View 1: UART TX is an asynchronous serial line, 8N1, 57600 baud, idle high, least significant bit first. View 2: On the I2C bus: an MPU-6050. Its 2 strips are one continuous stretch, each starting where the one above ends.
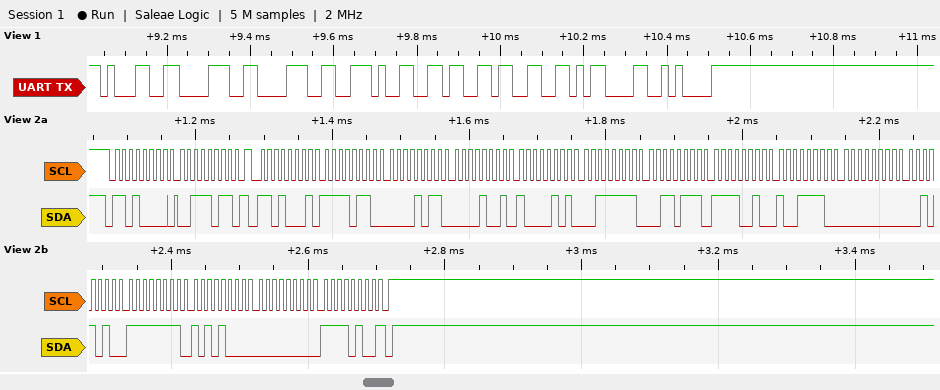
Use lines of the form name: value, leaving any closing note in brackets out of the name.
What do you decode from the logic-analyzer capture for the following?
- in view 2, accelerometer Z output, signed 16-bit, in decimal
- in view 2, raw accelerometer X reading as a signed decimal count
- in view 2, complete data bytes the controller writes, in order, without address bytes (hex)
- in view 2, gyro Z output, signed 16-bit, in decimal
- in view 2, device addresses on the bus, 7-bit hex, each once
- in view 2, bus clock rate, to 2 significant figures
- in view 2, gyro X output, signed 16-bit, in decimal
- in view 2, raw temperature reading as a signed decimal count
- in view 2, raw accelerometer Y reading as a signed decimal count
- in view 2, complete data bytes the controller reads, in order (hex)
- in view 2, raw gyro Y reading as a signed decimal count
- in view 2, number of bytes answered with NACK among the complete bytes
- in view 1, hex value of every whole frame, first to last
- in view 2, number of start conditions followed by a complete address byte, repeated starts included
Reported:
in view 2, accelerometer Z output, signed 16-bit, in decimal: 16183
in view 2, raw accelerometer X reading as a signed decimal count: -2549
in view 2, complete data bytes the controller writes, in order, without address bytes: 3B
in view 2, gyro Z output, signed 16-bit, in decimal: 244
in view 2, device addresses on the bus, 7-bit hex, each once: 0x68
in view 2, bus clock rate, to 2 significant figures: 100 kHz
in view 2, gyro X output, signed 16-bit, in decimal: 42
in view 2, raw temperature reading as a signed decimal count: -3426
in view 2, raw accelerometer Y reading as a signed decimal count: 2437
in view 2, complete data bytes the controller reads, in order: F6 0B 09 85 3F 37 F2 9E 00 2A FF A8 00 F4
in view 2, raw gyro Y reading as a signed decimal count: -88
in view 2, number of bytes answered with NACK among the complete bytes: 1
in view 1, hex value of every whole frame, first to last: 0x31 0x38 0x38 0x2E 0x36 0x33 0x0D 0x0A
in view 2, number of start conditions followed by a complete address byte, repeated starts included: 2
